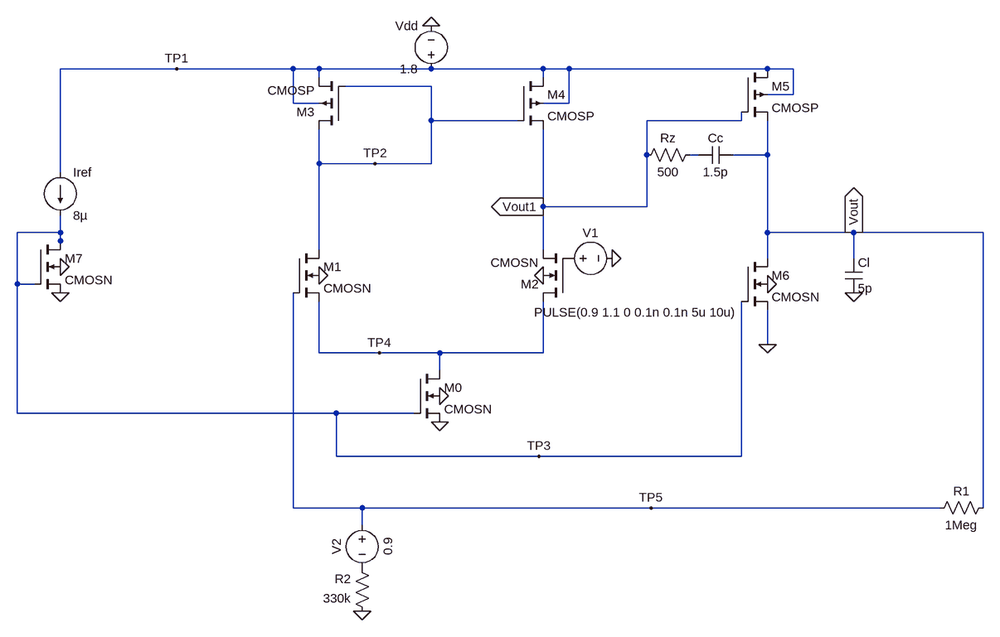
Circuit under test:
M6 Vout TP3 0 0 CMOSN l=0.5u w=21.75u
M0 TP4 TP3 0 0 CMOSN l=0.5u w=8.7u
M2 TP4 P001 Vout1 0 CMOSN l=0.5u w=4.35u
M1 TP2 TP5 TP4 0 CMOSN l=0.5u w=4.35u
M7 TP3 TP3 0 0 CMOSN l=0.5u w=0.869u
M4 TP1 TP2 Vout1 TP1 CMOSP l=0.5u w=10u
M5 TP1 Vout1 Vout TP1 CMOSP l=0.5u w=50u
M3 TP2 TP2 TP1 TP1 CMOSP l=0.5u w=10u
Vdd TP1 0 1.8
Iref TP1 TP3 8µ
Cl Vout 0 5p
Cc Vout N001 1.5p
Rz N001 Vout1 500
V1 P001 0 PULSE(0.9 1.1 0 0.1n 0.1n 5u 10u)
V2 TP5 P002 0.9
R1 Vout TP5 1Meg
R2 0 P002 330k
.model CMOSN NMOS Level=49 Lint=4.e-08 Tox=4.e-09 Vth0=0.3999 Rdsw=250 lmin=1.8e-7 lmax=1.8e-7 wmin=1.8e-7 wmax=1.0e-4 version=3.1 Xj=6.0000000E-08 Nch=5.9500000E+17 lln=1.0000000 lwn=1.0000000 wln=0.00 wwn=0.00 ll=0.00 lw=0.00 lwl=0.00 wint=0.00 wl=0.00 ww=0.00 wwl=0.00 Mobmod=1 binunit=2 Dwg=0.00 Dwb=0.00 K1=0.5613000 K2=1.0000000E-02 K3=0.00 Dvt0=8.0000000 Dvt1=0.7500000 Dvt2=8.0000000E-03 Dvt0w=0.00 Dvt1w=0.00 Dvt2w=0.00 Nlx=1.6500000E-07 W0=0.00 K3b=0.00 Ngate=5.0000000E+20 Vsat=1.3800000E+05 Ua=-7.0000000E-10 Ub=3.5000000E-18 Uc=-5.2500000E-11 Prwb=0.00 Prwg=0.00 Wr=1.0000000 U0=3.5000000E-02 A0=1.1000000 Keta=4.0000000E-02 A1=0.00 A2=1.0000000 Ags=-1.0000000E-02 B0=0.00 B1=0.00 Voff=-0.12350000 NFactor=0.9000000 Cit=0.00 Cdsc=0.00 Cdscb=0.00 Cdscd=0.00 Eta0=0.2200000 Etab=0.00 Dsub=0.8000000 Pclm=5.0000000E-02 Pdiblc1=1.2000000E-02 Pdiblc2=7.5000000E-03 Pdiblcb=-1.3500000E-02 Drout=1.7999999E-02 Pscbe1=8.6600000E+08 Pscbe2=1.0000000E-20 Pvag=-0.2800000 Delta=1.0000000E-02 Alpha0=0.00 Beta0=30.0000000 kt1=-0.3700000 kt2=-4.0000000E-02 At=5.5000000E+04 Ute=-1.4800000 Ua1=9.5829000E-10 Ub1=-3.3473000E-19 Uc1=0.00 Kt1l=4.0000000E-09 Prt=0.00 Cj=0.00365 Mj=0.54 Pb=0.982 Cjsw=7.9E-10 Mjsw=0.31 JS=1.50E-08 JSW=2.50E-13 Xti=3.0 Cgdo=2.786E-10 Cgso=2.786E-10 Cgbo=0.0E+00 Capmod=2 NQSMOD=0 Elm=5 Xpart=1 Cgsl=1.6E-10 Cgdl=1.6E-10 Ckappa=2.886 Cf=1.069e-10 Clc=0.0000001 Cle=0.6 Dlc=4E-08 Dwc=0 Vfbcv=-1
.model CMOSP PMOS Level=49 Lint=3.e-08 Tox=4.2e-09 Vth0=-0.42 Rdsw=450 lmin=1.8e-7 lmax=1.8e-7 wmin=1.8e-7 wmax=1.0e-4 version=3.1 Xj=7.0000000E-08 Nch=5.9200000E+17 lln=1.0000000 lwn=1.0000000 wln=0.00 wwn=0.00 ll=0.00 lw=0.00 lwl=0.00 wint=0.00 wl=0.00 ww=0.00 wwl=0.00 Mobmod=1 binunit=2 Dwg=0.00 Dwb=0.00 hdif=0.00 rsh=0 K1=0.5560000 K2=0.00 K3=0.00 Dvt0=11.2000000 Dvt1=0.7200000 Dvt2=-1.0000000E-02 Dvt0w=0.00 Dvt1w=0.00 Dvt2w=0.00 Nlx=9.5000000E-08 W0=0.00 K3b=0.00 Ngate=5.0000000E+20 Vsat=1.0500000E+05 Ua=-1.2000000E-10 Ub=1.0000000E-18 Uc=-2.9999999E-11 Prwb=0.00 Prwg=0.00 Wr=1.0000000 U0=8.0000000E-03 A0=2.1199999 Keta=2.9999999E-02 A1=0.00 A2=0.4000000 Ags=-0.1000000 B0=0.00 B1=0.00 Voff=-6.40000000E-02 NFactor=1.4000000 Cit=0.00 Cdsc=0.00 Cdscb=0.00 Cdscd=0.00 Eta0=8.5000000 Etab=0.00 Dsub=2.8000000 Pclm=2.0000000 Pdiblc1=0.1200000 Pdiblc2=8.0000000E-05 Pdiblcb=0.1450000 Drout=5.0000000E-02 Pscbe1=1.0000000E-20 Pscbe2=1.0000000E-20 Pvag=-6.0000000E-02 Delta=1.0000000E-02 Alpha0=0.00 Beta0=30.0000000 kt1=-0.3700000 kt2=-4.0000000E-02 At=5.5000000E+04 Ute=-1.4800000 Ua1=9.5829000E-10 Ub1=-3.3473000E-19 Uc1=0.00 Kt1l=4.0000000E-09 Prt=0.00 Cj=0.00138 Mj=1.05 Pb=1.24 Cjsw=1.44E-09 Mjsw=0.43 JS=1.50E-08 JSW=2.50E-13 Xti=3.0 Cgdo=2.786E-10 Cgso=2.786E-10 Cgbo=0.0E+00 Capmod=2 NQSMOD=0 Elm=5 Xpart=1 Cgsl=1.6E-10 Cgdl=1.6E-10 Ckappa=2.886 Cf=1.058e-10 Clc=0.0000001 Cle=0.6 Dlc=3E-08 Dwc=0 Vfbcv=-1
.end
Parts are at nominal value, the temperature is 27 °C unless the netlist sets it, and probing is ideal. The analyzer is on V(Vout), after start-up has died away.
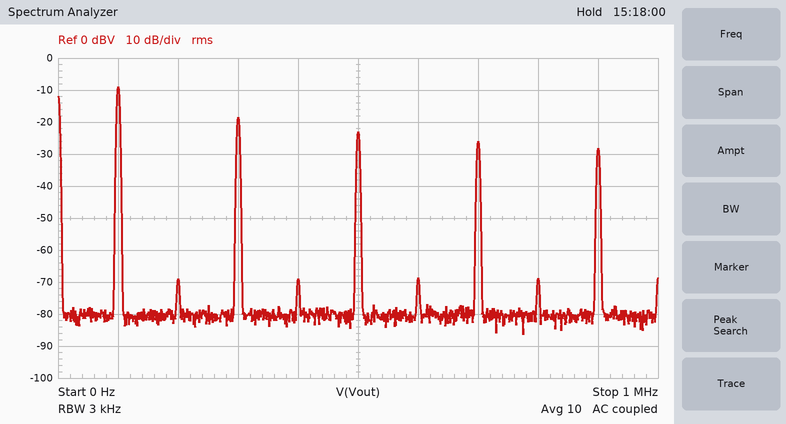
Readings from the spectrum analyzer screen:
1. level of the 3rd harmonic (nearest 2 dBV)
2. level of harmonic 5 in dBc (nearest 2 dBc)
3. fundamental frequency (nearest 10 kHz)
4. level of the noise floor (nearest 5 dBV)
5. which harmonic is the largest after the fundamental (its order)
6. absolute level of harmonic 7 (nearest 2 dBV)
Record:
-18 dBV
-14 dBc
100 kHz
-80 dBV
3
-26 dBV
